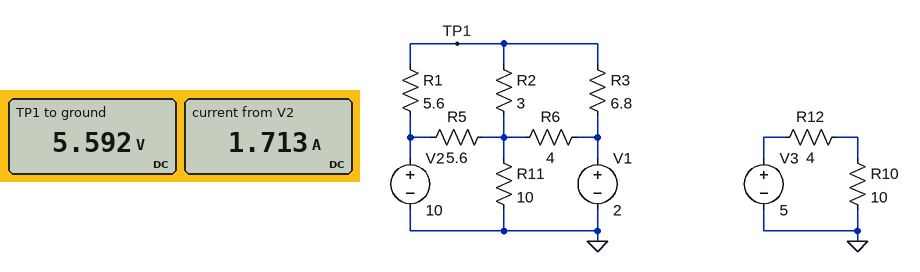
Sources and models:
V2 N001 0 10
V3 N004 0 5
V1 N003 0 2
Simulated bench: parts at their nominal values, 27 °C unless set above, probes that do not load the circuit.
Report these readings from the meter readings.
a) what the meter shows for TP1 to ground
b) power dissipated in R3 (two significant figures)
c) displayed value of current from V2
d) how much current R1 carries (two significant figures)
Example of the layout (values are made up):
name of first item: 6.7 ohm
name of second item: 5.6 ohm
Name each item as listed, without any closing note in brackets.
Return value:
what the meter shows for TP1 to ground: 5.592 V
power dissipated in R3: 1.9 W
displayed value of current from V2: 1.713 A
how much current R1 carries: 790 mA
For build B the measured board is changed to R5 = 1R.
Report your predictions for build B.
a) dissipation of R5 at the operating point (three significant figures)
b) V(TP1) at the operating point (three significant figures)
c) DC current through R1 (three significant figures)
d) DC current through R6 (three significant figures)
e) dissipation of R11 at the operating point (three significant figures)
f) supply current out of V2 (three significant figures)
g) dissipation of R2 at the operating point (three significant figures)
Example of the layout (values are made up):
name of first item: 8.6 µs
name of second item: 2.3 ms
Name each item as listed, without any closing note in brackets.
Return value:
dissipation of R5 at the operating point: 5.63 W
V(TP1) at the operating point: 7.01 V
DC current through R1: 533 mA
DC current through R6: 1.41 A
dissipation of R11 at the operating point: 5.82 W
supply current out of V2: 2.91 A
dissipation of R2 at the operating point: 125 mW
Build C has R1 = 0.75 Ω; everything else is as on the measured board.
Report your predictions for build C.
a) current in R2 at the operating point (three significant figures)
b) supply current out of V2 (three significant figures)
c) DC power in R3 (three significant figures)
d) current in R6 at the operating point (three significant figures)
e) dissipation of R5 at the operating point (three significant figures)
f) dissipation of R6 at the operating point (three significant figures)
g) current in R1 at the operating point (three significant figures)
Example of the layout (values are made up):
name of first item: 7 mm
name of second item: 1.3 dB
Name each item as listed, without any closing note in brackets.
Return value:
current in R2 at the operating point: 877 mA
supply current out of V2: 2.57 A
DC power in R3: 6.43 W
current in R6 at the operating point: 996 mA
dissipation of R5 at the operating point: 2.88 W
dissipation of R6 at the operating point: 3.97 W
current in R1 at the operating point: 1.85 A
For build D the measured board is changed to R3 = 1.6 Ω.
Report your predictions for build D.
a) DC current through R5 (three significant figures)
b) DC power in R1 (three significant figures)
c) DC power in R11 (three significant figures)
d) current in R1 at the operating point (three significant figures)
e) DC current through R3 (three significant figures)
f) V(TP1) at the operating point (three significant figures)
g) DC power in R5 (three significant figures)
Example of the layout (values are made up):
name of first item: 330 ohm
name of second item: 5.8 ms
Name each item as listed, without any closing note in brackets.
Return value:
DC current through R5: 1.04 A
DC power in R1: 6.67 W
DC power in R11: 1.73 W
current in R1 at the operating point: 1.09 A
DC current through R3: 1.18 A
V(TP1) at the operating point: 3.89 V
DC power in R5: 6.10 W
